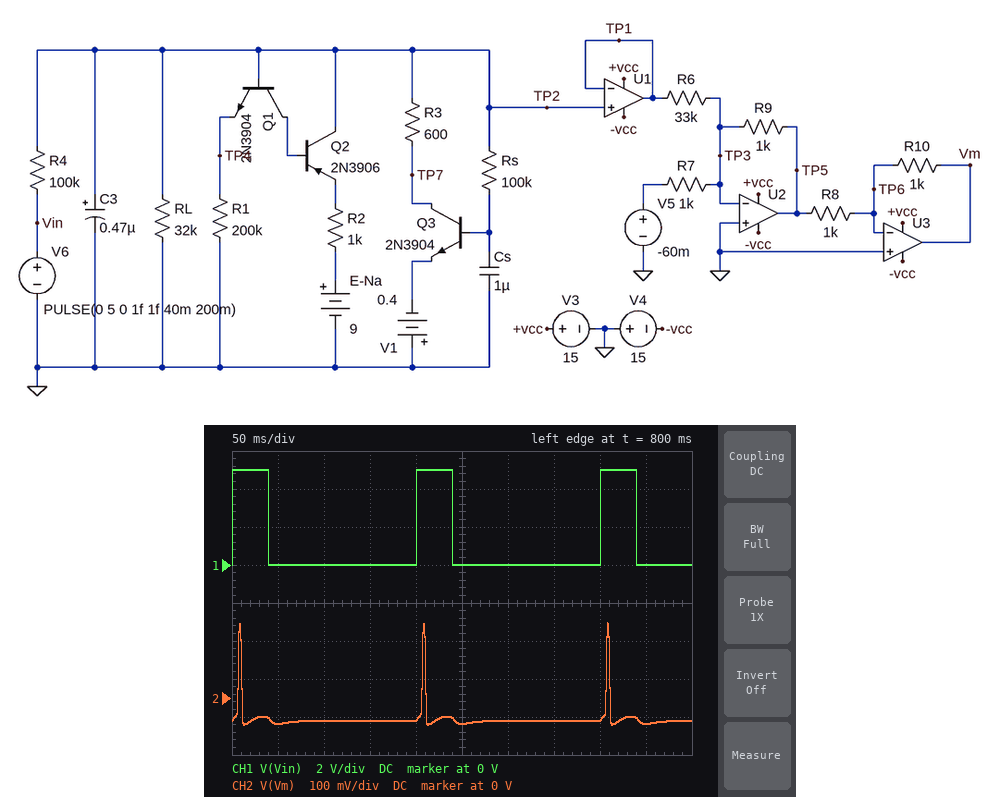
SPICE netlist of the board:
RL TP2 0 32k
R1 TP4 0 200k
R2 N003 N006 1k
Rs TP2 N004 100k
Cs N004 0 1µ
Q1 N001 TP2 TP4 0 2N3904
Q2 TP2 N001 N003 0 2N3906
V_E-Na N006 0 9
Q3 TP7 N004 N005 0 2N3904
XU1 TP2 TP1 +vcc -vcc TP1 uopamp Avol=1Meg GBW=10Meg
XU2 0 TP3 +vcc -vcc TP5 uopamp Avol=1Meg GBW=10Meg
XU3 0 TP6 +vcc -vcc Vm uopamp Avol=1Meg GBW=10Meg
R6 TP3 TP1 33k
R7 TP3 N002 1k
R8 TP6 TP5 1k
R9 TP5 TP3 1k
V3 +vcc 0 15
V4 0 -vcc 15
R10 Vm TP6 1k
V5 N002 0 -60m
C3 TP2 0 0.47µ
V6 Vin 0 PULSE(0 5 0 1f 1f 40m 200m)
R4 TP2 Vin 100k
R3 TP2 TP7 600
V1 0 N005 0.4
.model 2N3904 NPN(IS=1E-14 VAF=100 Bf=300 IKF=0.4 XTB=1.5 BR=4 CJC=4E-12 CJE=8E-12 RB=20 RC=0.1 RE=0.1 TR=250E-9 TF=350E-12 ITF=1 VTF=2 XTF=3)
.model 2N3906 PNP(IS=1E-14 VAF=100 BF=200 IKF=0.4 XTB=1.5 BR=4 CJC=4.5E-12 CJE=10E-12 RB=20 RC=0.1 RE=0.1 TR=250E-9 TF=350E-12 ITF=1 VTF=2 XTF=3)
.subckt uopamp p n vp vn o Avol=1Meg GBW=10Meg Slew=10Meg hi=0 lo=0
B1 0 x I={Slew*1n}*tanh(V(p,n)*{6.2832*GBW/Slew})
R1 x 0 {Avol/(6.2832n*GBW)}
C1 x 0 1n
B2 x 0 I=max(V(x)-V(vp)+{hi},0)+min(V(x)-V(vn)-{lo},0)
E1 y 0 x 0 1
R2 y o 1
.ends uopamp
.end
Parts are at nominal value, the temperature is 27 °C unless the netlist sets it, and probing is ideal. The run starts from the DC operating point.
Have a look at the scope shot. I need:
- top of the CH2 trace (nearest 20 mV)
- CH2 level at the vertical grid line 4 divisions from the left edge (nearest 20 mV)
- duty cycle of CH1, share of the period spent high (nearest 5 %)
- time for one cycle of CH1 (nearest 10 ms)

200 mV
-60 mV
20 %
200 ms
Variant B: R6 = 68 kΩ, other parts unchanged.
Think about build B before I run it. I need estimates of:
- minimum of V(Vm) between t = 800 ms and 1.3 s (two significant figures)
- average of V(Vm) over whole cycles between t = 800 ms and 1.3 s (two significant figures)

-65 mV
-58 mV
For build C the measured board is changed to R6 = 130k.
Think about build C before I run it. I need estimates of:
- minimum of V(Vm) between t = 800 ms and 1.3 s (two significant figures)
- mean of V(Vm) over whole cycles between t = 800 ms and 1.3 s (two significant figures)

-63 mV
-59 mV
